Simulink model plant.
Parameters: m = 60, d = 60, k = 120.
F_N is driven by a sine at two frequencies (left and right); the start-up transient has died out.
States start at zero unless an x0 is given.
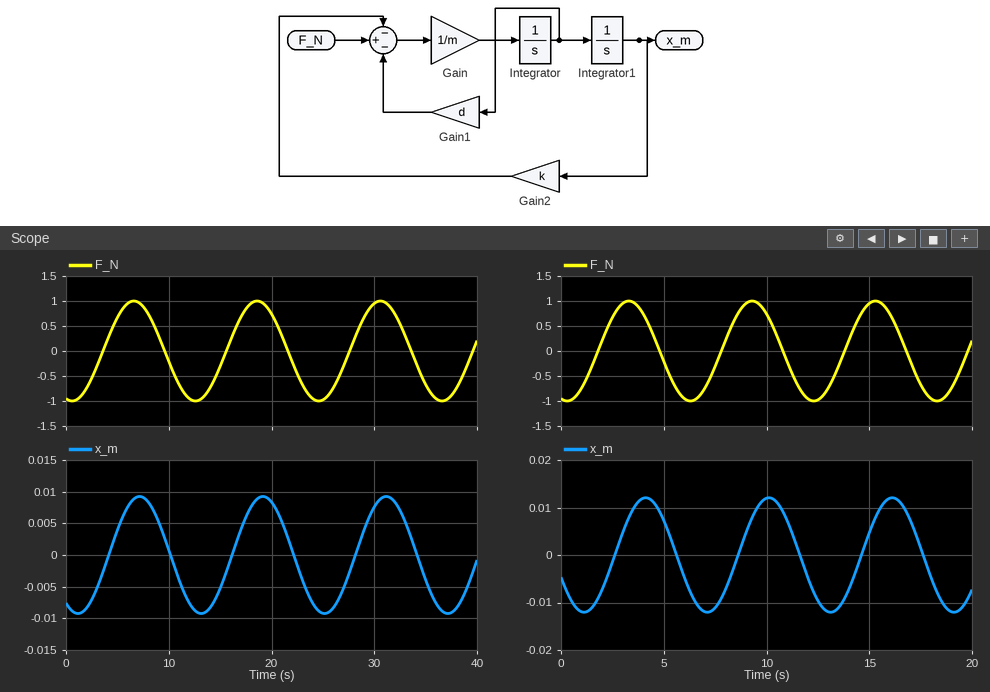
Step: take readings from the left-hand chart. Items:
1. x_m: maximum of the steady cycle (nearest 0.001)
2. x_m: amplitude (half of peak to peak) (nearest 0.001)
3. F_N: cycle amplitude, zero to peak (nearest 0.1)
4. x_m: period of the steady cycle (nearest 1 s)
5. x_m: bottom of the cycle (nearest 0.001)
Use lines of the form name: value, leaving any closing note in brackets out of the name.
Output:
x_m: maximum of the steady cycle: 0.009
x_m: amplitude (half of peak to peak): 0.009
F_N: cycle amplitude, zero to peak: 1.0
x_m: period of the steady cycle: 12 s
x_m: bottom of the cycle: -0.009
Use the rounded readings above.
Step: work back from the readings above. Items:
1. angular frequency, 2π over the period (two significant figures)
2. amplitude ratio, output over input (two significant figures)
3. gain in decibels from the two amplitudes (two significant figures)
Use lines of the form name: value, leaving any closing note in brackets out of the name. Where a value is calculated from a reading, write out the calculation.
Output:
angular frequency, 2π over the period: 2π / 12 = 0.52 rad/s
amplitude ratio, output over input: 0.009 / 1 = 0.0090
gain in decibels from the two amplitudes: 20 log10(0.009 / 1) = -41 dB
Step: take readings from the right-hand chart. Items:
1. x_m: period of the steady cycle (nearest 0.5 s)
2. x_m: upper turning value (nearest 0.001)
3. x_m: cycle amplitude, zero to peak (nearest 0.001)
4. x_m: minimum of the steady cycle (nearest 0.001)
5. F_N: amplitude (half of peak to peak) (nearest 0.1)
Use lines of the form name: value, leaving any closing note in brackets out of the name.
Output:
x_m: period of the steady cycle: 6.0 s
x_m: upper turning value: 0.012
x_m: cycle amplitude, zero to peak: 0.012
x_m: minimum of the steady cycle: -0.012
F_N: amplitude (half of peak to peak): 1.0
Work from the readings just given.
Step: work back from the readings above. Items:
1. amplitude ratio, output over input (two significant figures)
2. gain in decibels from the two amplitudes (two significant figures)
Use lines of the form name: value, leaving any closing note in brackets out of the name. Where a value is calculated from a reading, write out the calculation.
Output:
amplitude ratio, output over input: 0.012 / 1 = 0.012
gain in decibels from the two amplitudes: 20 log10(0.012 / 1) = -38 dB
